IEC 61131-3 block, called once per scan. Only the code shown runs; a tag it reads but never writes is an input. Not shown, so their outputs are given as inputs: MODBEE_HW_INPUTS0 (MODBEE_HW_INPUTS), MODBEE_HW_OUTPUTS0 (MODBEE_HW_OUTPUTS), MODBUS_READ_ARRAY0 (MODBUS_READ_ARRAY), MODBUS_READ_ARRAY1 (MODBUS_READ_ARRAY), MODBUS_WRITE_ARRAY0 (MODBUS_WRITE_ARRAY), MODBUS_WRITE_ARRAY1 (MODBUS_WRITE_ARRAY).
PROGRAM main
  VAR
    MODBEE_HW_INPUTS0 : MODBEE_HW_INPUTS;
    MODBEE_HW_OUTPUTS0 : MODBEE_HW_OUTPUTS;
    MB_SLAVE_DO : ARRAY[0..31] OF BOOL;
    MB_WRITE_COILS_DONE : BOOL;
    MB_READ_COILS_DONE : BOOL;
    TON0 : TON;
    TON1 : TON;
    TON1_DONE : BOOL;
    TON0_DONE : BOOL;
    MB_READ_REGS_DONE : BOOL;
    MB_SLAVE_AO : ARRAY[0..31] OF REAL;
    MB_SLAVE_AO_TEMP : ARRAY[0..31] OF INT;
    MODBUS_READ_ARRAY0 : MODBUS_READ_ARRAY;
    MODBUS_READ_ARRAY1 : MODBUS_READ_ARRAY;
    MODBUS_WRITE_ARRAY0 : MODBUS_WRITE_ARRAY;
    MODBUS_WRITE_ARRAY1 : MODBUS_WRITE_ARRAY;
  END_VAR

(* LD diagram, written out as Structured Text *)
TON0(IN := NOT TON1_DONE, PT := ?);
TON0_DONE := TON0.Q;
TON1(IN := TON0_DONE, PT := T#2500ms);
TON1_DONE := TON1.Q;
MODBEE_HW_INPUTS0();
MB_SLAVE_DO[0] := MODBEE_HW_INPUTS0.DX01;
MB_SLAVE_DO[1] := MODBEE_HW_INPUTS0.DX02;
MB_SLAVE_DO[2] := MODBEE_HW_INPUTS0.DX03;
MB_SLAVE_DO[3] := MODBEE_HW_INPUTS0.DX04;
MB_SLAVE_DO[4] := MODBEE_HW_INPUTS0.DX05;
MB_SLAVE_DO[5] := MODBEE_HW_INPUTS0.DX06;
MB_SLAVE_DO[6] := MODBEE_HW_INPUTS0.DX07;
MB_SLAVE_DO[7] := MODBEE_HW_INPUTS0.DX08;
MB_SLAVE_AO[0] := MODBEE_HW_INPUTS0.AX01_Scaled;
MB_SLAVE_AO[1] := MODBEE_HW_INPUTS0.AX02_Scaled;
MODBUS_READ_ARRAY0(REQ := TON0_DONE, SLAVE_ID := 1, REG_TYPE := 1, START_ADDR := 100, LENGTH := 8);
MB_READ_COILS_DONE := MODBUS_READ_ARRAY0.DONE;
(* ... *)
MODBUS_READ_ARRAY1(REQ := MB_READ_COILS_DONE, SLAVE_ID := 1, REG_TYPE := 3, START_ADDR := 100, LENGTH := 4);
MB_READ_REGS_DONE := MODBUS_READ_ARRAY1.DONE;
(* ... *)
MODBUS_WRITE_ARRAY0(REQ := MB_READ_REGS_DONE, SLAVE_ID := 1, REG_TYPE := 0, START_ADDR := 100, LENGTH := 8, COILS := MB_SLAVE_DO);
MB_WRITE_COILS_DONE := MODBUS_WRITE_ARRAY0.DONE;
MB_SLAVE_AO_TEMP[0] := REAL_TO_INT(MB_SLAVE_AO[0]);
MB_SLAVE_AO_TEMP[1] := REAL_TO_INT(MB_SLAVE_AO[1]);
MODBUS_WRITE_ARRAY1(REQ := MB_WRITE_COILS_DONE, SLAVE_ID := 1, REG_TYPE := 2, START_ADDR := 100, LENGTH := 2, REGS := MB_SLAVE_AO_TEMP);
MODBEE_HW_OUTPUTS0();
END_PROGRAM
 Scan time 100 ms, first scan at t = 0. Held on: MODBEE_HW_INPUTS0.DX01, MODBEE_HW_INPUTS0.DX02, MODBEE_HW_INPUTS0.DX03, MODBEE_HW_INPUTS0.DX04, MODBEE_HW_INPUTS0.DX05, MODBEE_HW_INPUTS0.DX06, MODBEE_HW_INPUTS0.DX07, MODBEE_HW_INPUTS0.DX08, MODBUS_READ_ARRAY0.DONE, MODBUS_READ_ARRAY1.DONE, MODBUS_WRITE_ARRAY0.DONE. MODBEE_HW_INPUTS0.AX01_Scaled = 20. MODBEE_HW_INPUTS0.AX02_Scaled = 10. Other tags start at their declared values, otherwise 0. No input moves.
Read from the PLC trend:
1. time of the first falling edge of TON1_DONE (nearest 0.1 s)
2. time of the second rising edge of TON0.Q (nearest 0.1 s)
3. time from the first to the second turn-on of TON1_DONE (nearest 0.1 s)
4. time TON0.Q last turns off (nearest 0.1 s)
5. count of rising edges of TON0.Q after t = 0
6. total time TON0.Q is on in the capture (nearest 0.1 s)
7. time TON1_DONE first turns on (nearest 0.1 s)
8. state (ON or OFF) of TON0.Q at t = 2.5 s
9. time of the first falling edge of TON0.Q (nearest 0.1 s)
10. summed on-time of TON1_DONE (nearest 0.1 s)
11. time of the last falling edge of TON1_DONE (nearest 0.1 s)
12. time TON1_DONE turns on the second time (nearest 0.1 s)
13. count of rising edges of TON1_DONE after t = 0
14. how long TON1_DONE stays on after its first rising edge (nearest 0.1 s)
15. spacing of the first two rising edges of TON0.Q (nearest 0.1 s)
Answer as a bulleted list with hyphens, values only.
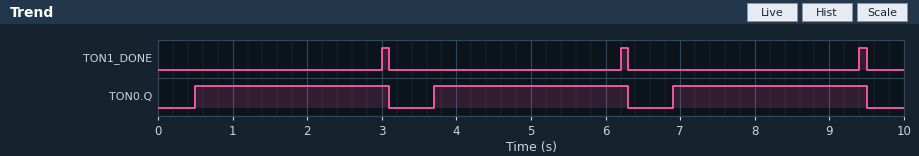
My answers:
- 3.1 s
- 3.7 s
- 3.2 s
- 9.5 s
- 3
- 7.8 s
- 3.0 s
- ON
- 3.1 s
- 0.3 s
- 9.5 s
- 6.2 s
- 3
- 0.1 s
- 3.2 s
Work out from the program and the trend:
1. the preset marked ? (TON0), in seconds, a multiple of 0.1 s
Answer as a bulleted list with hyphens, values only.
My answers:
- 0.5 s
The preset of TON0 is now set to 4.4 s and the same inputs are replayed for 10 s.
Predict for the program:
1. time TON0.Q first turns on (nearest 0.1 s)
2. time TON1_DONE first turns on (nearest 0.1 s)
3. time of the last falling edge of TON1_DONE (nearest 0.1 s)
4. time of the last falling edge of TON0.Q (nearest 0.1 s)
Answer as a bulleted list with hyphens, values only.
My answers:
- 4.4 s
- 6.9 s
- 7.0 s
- 7.0 s
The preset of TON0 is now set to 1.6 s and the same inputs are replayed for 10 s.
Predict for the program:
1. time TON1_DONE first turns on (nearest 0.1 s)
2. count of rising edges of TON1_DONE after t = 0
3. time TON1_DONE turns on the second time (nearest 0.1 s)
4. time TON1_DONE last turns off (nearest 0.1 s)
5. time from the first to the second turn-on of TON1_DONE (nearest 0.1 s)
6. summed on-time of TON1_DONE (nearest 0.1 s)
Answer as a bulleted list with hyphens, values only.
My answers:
- 4.1 s
- 2
- 8.4 s
- 8.5 s
- 4.3 s
- 0.2 s
